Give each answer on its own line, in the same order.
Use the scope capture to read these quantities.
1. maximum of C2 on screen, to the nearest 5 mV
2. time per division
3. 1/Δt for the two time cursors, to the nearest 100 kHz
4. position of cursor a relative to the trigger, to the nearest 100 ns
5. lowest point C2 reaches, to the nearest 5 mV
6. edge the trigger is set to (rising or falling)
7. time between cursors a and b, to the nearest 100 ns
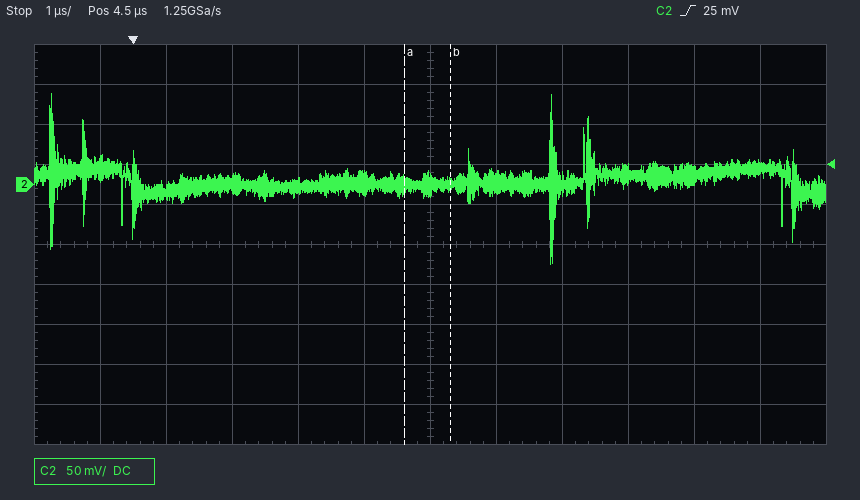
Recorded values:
115 mV
1 µs
1.4 MHz
+4.1 µs
-100 mV
rising
700 ns
